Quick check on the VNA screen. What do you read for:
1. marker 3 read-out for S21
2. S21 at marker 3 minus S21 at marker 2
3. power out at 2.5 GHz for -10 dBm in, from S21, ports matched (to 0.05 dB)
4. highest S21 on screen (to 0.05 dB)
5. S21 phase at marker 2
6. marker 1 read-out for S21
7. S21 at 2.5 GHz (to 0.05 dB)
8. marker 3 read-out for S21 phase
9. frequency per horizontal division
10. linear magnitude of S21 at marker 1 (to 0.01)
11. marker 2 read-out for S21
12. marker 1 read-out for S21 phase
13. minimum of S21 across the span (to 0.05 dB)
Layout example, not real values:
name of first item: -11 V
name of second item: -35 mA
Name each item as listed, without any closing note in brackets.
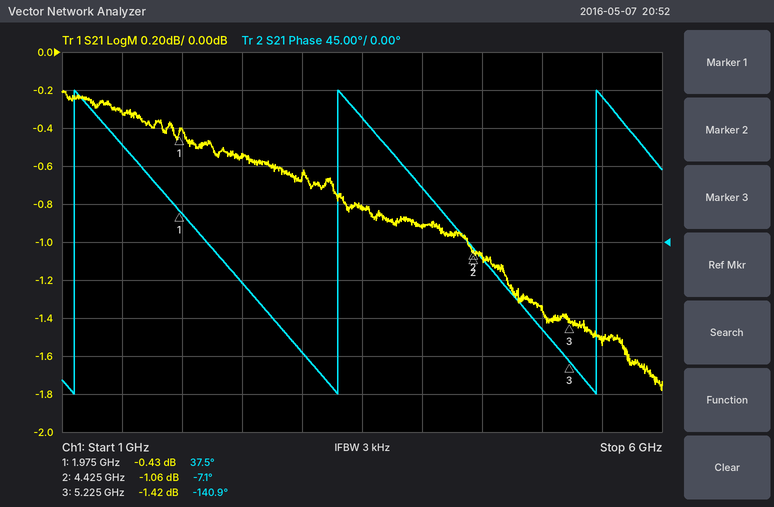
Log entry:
marker 3 read-out for S21: -1.42 dB
S21 at marker 3 minus S21 at marker 2: -0.36 dB
power out at 2.5 GHz for -10 dBm in, from S21, ports matched: -10.55 dBm
highest S21 on screen: -0.20 dB
S21 phase at marker 2: -7.1°
marker 1 read-out for S21: -0.43 dB
S21 at 2.5 GHz: -0.55 dB
marker 3 read-out for S21 phase: -140.9°
frequency per horizontal division: 500 MHz
linear magnitude of S21 at marker 1: 0.95
marker 2 read-out for S21: -1.06 dB
marker 1 read-out for S21 phase: 37.5°
minimum of S21 across the span: -1.80 dB
